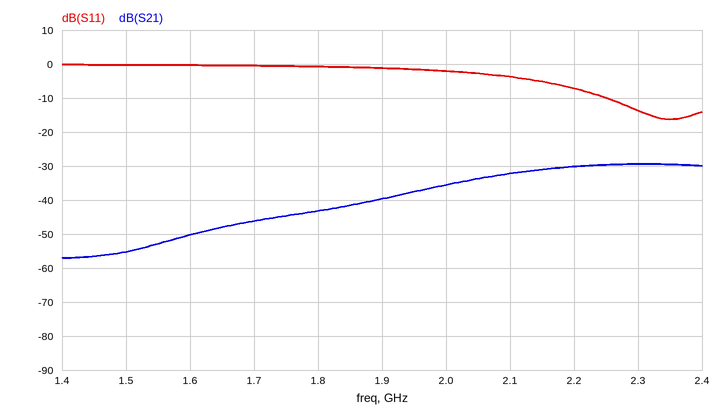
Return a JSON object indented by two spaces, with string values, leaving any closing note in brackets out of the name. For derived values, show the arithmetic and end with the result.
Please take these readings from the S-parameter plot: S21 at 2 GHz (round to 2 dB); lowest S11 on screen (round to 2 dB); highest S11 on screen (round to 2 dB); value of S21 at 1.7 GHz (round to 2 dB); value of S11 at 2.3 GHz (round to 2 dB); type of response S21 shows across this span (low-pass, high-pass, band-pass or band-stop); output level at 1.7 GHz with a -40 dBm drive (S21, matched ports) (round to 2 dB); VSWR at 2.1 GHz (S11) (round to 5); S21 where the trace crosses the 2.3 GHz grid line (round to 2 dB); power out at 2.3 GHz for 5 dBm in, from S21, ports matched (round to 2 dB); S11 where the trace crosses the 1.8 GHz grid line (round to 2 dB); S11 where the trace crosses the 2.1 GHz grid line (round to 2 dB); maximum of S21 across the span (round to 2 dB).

{
  "S21 at 2 GHz": "-36 dB",
  "lowest S11 on screen": "-16 dB",
  "highest S11 on screen": "0 dB",
  "value of S21 at 1.7 GHz": "-46 dB",
  "value of S11 at 2.3 GHz": "-14 dB",
  "type of response S21 shows across this span": "high-pass",
  "output level at 1.7 GHz with a -40 dBm drive (S21, matched ports)": "-40 dBm + (-46 dB) = -86 dBm",
  "VSWR at 2.1 GHz (S11)": "|Γ| = 10^(-4/20) = 0.6310; VSWR = (1 + 0.6310)/(1 − 0.6310) ≈ 4.42, so 5 to the nearest 5",
  "S21 where the trace crosses the 2.3 GHz grid line": "-30 dB",
  "power out at 2.3 GHz for 5 dBm in, from S21, ports matched": "5 dBm + (-30 dB) = -24 dBm",
  "S11 where the trace crosses the 1.8 GHz grid line": "0 dB",
  "S11 where the trace crosses the 2.1 GHz grid line": "-4 dB",
  "maximum of S21 across the span": "-30 dB"
}
